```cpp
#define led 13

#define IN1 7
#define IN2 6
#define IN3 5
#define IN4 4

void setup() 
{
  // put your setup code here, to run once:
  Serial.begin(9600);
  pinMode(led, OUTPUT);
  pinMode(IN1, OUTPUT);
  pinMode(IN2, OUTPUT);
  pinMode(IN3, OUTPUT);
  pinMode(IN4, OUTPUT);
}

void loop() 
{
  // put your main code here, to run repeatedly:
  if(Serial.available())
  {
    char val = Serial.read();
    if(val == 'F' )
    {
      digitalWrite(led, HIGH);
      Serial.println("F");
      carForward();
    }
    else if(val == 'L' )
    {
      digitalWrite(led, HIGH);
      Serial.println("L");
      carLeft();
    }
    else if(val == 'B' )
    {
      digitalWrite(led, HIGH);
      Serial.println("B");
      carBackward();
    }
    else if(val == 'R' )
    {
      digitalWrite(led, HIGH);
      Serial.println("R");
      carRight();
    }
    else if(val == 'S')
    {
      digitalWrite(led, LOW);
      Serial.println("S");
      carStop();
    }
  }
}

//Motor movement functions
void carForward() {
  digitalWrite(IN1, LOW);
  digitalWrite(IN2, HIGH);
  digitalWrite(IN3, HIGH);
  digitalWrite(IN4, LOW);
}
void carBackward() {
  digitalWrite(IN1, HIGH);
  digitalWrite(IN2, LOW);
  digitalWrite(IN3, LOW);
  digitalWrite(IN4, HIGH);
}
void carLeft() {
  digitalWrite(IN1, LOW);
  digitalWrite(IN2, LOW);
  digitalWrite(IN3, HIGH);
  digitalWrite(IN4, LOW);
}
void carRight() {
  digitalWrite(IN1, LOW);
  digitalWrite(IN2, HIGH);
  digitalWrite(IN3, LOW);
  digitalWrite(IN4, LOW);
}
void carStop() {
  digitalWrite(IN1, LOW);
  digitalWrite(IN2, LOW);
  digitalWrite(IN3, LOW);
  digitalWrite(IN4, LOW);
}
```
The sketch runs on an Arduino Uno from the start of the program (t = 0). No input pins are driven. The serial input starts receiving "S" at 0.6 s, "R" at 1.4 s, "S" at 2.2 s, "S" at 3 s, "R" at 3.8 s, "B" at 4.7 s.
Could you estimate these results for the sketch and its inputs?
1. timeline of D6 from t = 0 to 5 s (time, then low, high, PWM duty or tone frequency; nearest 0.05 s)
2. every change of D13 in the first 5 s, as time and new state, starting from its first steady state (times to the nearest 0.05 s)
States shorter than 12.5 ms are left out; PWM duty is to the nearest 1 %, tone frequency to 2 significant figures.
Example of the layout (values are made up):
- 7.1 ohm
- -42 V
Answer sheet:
- 0 s low; 1.4 s high; 2.2 s low; 3.8 s high; 4.7 s low
- 0 s low; 1.4 s high; 2.2 s low; 3.8 s high
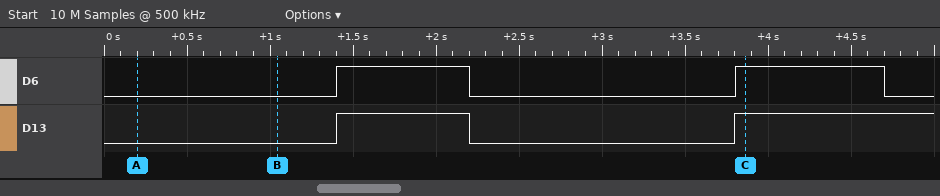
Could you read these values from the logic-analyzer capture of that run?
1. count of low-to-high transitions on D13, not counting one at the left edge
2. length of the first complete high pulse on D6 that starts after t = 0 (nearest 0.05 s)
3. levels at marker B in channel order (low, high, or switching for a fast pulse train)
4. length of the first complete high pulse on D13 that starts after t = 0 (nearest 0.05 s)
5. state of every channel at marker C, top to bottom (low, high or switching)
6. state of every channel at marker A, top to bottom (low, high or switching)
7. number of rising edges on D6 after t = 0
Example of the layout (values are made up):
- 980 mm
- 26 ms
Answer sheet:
- 2
- 0.80 s
- D6 low, D13 low
- 0.80 s
- D6 high, D13 high
- D6 low, D13 low
- 2
